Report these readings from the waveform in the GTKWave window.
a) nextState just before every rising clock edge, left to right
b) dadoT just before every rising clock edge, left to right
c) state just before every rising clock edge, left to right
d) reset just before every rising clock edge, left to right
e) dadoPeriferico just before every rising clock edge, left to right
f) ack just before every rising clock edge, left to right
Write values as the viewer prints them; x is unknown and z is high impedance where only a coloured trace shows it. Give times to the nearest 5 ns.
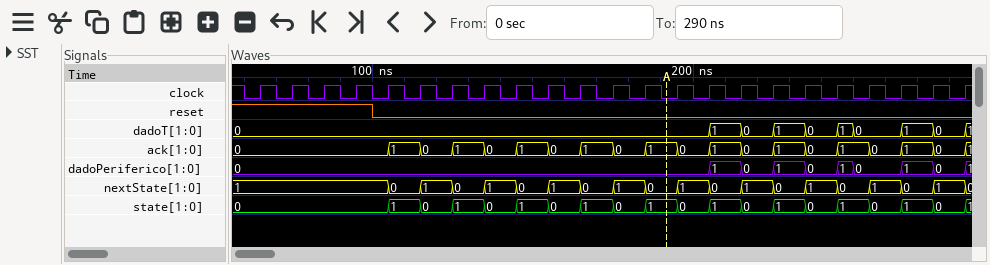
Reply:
1, 1, 1, 1, 1, 0, 1, 0, 1, 0, 1, 0, 1, 0, 1, 0, 1, 0, 1, 0, 1, 0, 1
0, 0, 0, 0, 0, 0, 0, 0, 0, 0, 0, 0, 0, 0, 0, 1, 0, 1, 0, 0, 0, 1, 0
0, 0, 0, 0, 0, 1, 0, 1, 0, 1, 0, 1, 0, 1, 0, 1, 0, 1, 0, 1, 0, 1, 0
1 1 1 1 0 0 0 0 0 0 0 0 0 0 0 0 0 0 0 0 0 0 0
0, 0, 0, 0, 0, 0, 0, 0, 0, 0, 0, 0, 0, 0, 0, 1, 0, 1, 0, 0, 0, 1, 0
0, 0, 0, 0, 0, 1, 0, 1, 0, 1, 0, 1, 0, 1, 0, 1, 0, 1, 0, 1, 0, 1, 0
